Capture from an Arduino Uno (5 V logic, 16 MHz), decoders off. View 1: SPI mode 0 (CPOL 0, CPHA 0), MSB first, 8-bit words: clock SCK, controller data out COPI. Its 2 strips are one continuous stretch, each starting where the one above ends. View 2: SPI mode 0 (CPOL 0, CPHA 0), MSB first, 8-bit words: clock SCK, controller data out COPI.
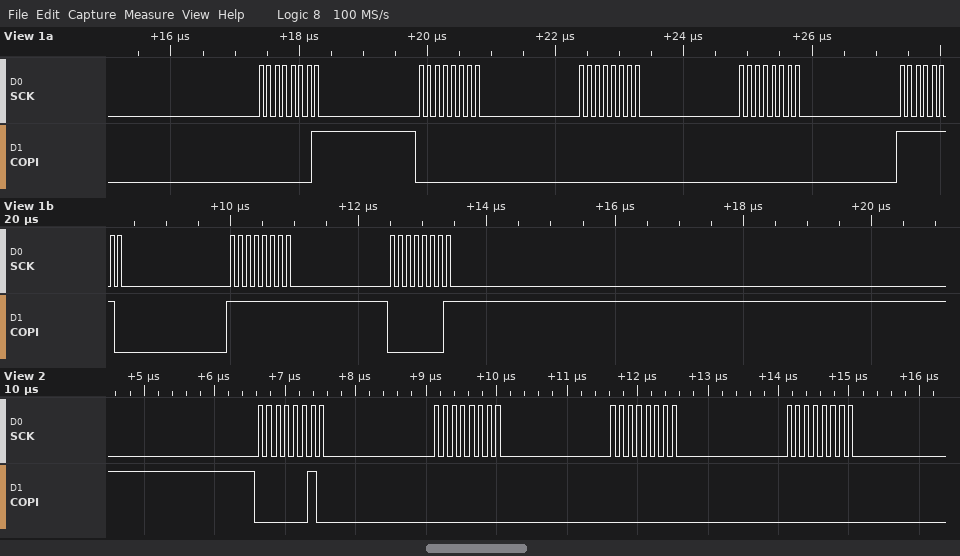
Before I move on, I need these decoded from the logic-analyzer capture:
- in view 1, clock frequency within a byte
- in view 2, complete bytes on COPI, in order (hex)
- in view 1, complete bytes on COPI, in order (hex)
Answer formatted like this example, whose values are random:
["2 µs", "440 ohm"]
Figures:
["8 MHz", "02 00 00 00", "01 00 00 00 FE FF 01"]
